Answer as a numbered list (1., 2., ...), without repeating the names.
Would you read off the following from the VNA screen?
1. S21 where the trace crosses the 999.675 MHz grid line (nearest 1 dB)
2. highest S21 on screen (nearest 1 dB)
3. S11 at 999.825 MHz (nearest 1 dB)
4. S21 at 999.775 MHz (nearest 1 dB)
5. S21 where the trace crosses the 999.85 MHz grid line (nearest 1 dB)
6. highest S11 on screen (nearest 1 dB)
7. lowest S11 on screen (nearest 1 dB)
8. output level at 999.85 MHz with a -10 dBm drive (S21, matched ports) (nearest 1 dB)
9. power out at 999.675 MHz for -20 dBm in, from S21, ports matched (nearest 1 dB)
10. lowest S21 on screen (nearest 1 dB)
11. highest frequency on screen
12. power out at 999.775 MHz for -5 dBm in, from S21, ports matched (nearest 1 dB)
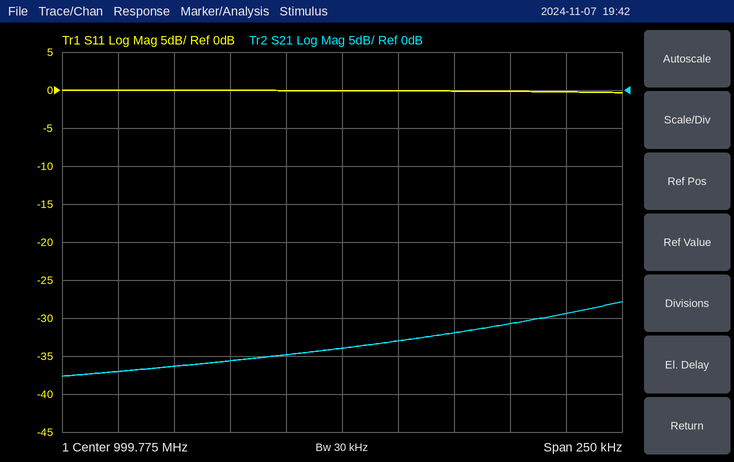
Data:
1. -37 dB
2. -28 dB
3. 0 dB
4. -34 dB
5. -31 dB
6. 0 dB
7. 0 dB
8. -41 dBm
9. -57 dBm
10. -38 dB
11. 999.9 MHz
12. -39 dBm
